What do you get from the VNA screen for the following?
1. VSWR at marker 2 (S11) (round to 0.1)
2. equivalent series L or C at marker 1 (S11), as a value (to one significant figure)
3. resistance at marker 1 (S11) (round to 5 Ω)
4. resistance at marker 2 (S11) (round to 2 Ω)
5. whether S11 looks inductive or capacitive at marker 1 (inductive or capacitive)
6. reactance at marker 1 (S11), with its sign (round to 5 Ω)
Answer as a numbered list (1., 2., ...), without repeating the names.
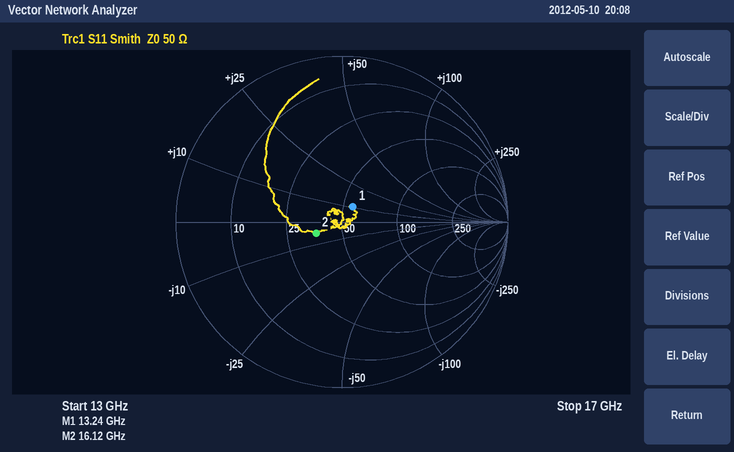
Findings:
1. 1.4
2. 100 pH
3. 55 Ω
4. 36 Ω
5. inductive
6. +10 Ω
